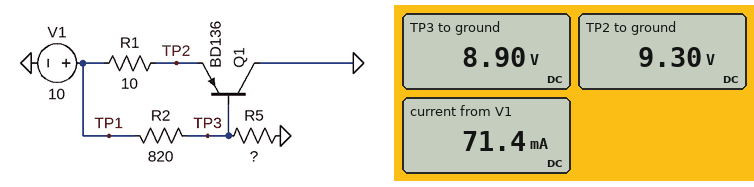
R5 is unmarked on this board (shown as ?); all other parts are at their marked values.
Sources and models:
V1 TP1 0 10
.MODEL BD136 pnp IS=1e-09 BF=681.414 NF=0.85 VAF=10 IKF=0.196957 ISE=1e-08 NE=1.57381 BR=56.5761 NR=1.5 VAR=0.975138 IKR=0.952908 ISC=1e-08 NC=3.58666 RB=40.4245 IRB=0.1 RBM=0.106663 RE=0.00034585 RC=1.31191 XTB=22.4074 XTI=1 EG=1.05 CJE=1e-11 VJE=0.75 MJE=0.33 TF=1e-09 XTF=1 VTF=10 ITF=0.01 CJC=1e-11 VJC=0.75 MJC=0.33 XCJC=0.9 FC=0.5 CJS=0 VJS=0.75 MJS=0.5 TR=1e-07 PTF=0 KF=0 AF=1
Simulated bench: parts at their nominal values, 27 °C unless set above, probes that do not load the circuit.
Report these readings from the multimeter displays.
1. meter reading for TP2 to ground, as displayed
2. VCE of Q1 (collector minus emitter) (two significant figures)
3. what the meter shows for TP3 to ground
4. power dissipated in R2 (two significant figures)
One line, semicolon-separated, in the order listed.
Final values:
9.30 V; -9.3 V; 8.90 V; 1.5 mW
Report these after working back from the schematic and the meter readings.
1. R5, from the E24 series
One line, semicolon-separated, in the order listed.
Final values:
5.6 kΩ
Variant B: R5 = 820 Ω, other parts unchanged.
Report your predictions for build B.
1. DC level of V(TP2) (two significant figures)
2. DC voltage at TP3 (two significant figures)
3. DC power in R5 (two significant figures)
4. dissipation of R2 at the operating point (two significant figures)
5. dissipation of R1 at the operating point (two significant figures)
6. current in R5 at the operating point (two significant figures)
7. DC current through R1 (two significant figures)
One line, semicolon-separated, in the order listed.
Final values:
6.4 V; 5.8 V; 41 mW; 21 mW; 1.3 W; 7.1 mA; 360 mA
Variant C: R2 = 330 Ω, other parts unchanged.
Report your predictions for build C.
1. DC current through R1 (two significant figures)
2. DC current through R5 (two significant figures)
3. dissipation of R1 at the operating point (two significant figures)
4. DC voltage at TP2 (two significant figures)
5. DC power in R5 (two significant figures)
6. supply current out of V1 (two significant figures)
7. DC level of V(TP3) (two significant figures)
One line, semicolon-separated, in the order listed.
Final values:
17 mA; 1.7 mA; 2.9 mW; 9.8 V; 16 mW; 19 mA; 9.5 V
